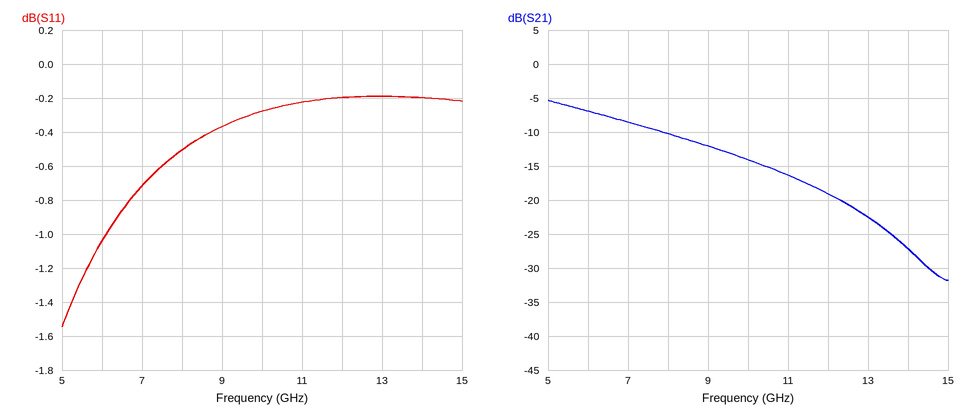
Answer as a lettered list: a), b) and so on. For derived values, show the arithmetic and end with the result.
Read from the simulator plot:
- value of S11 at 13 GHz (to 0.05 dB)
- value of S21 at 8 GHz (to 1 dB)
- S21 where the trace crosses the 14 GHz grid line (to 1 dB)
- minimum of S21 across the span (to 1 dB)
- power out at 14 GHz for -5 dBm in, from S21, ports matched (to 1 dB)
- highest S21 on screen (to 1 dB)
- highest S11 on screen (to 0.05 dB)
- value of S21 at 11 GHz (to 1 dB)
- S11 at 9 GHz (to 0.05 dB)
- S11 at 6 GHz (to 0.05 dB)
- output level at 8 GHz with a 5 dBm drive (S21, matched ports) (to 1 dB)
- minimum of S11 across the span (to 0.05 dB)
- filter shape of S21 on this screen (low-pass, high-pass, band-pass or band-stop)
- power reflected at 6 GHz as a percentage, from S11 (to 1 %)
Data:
a) -0.20 dB
b) -10 dB
c) -27 dB
d) -32 dB
e) -5 dBm + (-27 dB) = -32 dBm
f) -5 dB
g) -0.20 dB
h) -16 dB
i) -0.35 dB
j) -1.05 dB
k) 5 dBm + (-10 dB) = -5 dBm
l) -1.55 dB
m) low-pass
n) 10^(-1.05/10) ≈ 79 %
